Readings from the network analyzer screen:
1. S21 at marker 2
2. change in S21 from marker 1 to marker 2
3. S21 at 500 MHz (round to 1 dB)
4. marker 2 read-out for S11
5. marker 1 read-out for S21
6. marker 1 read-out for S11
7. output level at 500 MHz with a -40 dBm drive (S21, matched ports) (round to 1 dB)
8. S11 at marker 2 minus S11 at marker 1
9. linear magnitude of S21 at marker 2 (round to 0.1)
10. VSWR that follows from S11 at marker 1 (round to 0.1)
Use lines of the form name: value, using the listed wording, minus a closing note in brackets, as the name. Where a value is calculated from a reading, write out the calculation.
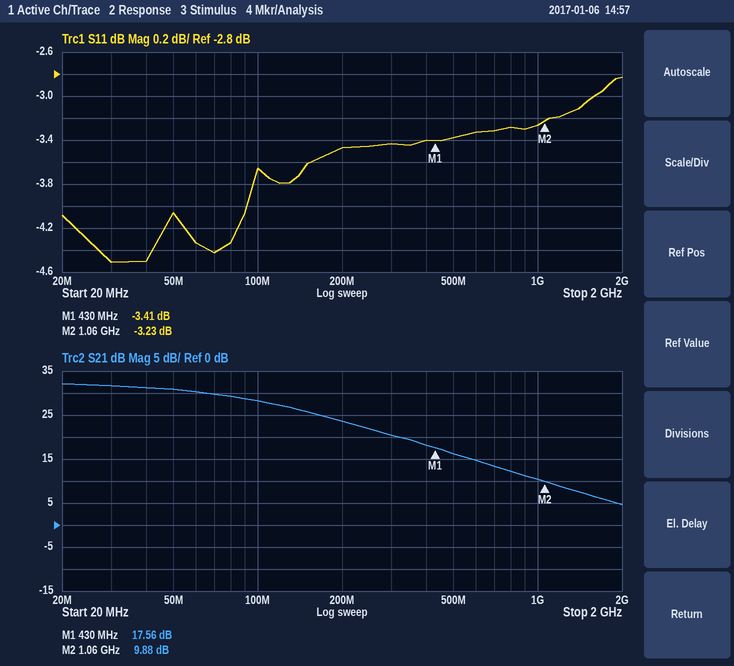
S21 at marker 2: 9.88 dB
change in S21 from marker 1 to marker 2: 9.88 − (17.56) = -7.68 dB
S21 at 500 MHz: 16 dB
marker 2 read-out for S11: -3.23 dB
marker 1 read-out for S21: 17.56 dB
marker 1 read-out for S11: -3.41 dB
output level at 500 MHz with a -40 dBm drive (S21, matched ports): -40 dBm + (16 dB) = -24 dBm
S11 at marker 2 minus S11 at marker 1: -3.23 − (-3.41) = 0.18 dB
linear magnitude of S21 at marker 2: 10^(9.88/20) ≈ 3.1
VSWR that follows from S11 at marker 1: (1 + 0.6753)/(1 − 0.6753) ≈ 5.2
